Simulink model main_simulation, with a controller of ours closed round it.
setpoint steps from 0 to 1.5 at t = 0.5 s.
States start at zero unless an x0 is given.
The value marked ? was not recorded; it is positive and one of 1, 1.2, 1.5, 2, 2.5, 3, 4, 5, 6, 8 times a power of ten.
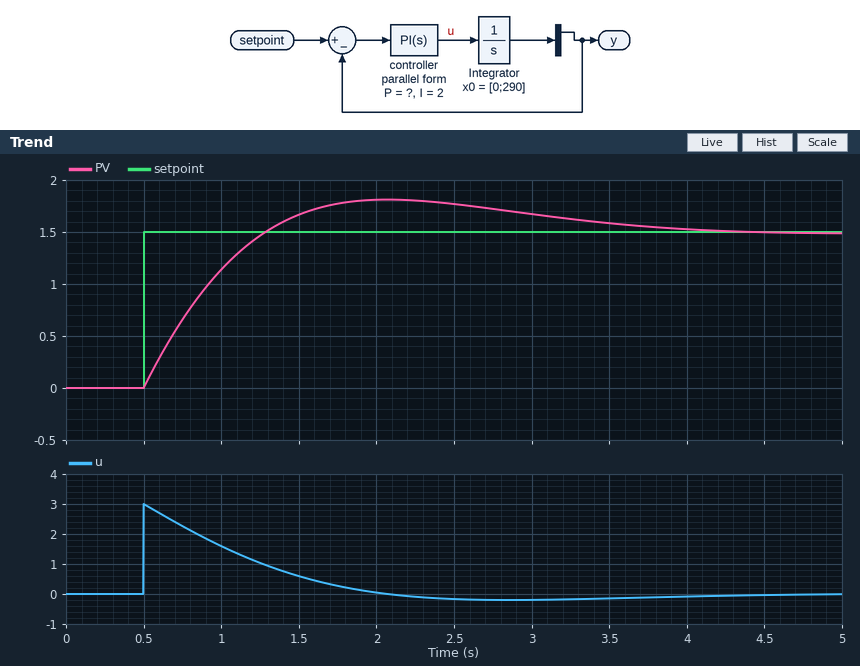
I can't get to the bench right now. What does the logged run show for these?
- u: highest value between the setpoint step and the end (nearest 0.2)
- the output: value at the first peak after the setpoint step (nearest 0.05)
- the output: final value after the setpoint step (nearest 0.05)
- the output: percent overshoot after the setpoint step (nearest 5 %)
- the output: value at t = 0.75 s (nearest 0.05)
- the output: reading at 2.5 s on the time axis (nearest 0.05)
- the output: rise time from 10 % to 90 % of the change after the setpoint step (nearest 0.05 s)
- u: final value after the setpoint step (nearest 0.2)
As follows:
3.0
1.80
1.50
20 %
0.65
1.75
0.60 s
0.0
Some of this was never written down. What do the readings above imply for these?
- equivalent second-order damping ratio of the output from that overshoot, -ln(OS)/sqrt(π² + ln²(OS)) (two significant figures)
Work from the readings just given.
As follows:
0.46
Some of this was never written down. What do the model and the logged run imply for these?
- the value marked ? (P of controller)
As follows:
2
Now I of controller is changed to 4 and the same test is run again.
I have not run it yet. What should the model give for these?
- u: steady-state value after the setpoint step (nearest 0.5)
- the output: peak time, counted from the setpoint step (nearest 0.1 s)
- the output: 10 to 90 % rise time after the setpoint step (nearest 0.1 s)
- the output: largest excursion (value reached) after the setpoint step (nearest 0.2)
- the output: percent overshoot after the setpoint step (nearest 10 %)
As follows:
0.0
1.2 s
0.5 s
2.0
30 %
